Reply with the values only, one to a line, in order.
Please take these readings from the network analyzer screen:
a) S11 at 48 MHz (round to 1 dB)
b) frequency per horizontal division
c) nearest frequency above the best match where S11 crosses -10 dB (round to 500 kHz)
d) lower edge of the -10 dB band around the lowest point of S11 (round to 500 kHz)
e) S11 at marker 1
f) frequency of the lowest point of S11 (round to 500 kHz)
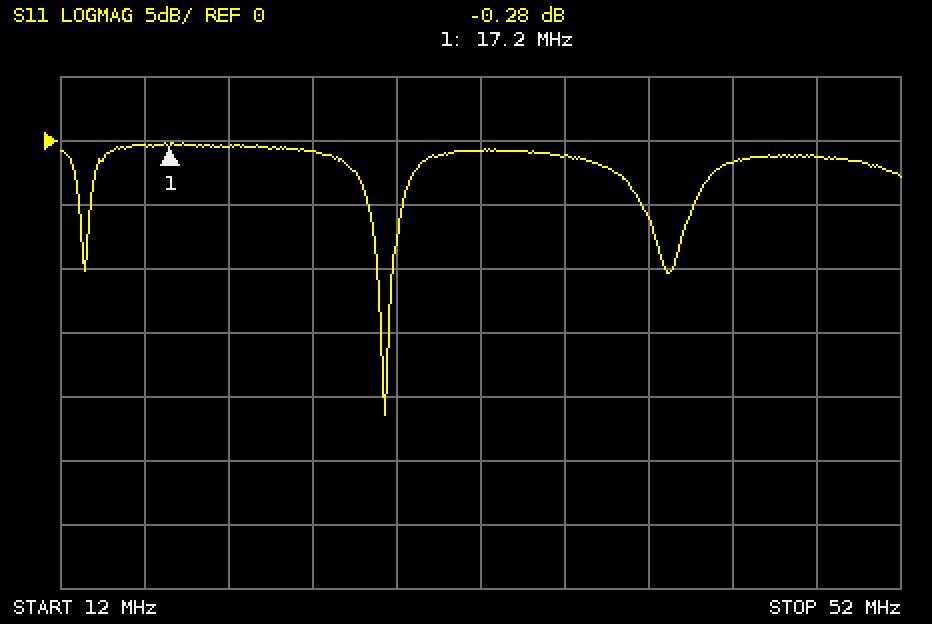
-1 dB
4 MHz
28.0 MHz
27.0 MHz
-0.28 dB
27.5 MHz
